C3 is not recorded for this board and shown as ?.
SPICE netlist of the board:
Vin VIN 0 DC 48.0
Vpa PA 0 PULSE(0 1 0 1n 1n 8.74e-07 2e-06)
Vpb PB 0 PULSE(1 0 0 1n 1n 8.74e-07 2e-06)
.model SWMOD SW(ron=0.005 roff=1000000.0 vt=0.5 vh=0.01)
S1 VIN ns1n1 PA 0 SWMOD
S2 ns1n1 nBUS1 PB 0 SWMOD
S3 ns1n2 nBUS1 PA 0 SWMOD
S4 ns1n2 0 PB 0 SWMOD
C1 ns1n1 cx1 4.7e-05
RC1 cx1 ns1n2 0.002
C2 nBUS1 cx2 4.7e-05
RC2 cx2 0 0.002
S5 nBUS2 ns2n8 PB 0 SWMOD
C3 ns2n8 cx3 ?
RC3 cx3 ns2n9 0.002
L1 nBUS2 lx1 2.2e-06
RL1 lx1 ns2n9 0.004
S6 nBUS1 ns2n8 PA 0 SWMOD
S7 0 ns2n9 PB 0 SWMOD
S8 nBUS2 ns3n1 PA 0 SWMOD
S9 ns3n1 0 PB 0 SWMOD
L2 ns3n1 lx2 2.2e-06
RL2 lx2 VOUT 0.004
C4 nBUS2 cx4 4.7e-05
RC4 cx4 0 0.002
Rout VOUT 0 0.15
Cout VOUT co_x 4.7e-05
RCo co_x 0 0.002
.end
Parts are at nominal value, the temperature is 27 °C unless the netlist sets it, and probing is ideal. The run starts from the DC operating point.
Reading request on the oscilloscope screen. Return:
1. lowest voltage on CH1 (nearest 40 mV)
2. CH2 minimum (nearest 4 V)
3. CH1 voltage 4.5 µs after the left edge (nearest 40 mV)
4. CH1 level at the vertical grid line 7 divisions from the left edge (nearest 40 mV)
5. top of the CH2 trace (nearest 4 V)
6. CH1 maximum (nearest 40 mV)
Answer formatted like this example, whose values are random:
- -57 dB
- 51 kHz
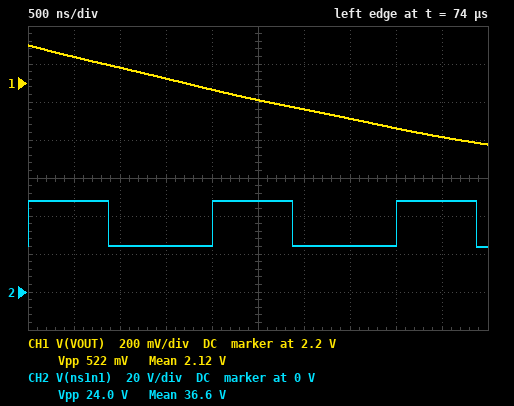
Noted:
- 1.88 V
- 24 V
- 1.92 V
- 2.00 V
- 48 V
- 2.40 V
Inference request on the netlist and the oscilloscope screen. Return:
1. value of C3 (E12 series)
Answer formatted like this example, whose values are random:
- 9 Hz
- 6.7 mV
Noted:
- 82 µF
